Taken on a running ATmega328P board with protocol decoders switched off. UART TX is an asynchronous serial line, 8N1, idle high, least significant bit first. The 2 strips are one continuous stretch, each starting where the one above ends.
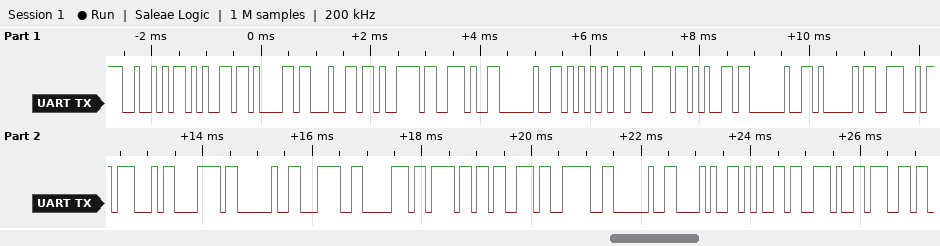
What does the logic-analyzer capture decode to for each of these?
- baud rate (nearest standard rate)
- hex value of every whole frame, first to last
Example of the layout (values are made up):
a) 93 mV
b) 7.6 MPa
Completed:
a) 9600 baud
b) 0x52 0x65 0x61 0x64 0x79 0x2E 0x20 0x55 0x73 0x65 0x20 0x41 0x4E 0x47 0x78 0x20 0x3C 0x70 0x6F 0x73 0x3E 0x20 0x28 0x65 0x2E 0x67
